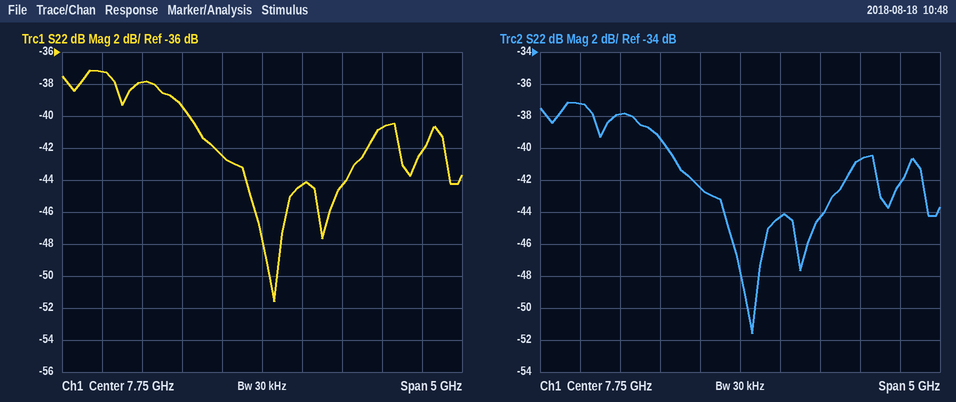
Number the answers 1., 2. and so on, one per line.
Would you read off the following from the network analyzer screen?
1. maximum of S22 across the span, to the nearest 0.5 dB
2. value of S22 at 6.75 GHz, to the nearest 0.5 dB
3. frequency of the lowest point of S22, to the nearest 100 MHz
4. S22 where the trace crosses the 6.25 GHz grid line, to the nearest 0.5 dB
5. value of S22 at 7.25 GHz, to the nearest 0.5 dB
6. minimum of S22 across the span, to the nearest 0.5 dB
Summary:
1. -37.0 dB
2. -39.5 dB
3. 7.9 GHz
4. -38.0 dB
5. -42.5 dB
6. -51.5 dB
